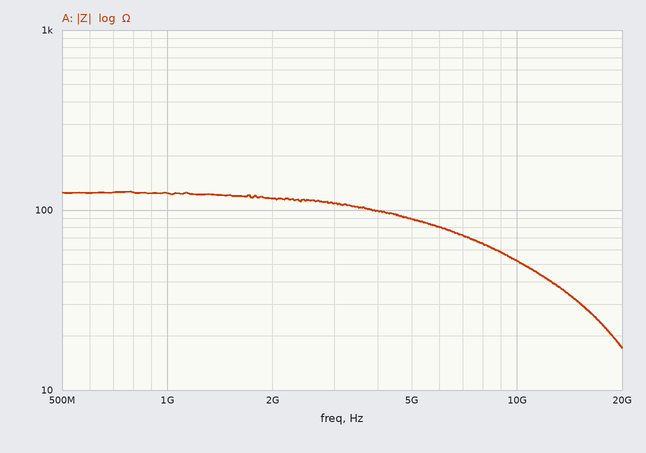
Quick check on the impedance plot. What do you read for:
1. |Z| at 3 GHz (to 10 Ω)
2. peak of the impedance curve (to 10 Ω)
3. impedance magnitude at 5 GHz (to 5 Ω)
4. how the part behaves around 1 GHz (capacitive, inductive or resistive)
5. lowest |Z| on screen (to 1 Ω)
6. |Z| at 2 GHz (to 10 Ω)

110 Ω
130 Ω
90 Ω
resistive
17 Ω
120 Ω
